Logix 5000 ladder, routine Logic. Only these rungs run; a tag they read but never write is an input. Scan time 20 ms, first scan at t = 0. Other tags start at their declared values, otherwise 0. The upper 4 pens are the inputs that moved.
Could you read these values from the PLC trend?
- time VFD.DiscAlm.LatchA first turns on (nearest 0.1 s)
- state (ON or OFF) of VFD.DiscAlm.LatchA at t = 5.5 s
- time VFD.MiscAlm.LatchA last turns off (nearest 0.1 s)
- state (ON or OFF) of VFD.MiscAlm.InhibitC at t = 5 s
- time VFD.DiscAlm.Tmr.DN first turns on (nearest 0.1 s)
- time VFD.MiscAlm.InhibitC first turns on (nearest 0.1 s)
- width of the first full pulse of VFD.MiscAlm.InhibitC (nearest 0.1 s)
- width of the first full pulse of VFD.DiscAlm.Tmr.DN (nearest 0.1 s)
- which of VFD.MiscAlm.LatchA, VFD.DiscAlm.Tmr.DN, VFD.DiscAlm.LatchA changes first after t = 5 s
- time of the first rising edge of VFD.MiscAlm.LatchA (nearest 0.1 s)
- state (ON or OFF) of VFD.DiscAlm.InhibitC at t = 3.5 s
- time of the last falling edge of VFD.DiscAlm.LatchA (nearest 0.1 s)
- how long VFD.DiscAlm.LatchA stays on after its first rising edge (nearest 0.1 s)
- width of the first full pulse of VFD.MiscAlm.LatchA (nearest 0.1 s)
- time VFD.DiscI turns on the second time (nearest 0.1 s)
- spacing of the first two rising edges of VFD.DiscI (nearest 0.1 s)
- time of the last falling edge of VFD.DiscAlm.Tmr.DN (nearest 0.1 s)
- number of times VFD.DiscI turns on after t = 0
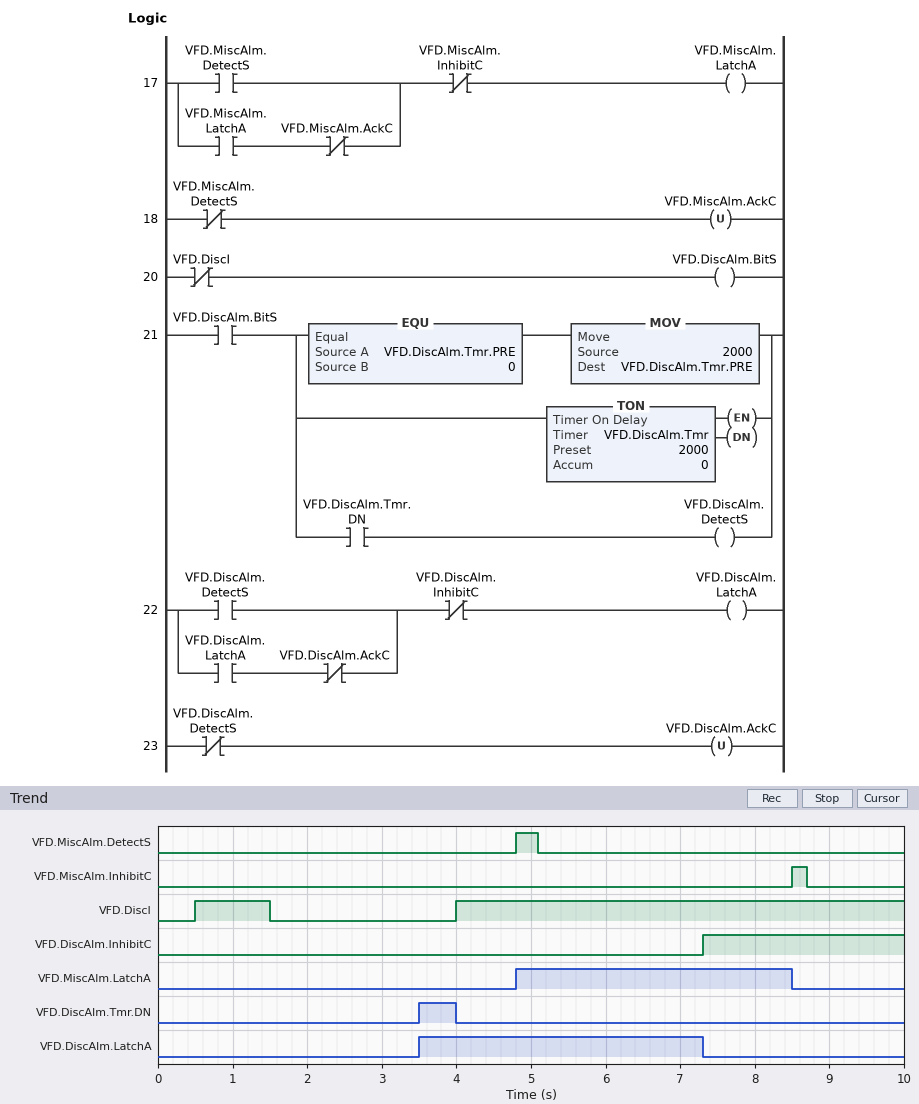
3.5 s
ON
8.5 s
OFF
3.5 s
8.5 s
0.2 s
0.5 s
VFD.DiscAlm.LatchA
4.8 s
OFF
7.3 s
3.8 s
3.7 s
4.0 s
3.5 s
4.0 s
2
